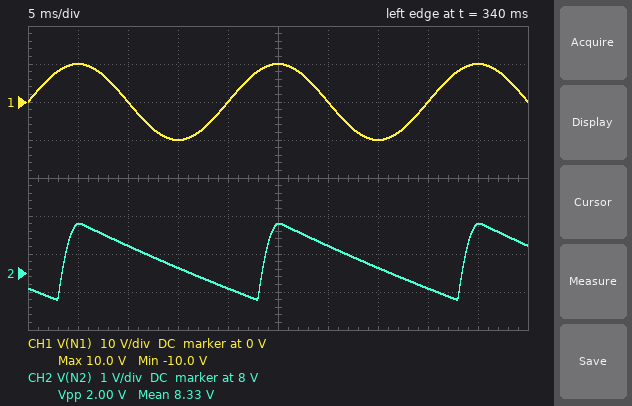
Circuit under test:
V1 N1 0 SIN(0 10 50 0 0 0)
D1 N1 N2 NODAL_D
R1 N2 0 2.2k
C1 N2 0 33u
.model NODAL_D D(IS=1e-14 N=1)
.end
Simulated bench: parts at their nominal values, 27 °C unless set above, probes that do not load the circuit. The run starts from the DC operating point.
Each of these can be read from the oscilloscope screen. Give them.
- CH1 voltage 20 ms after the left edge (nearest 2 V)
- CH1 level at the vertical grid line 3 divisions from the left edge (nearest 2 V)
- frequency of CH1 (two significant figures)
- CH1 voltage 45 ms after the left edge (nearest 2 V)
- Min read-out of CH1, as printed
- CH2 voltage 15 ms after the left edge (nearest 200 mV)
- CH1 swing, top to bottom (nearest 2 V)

0 V
-10 V
50 Hz
10 V
-10.0 V
8.2 V
20 V
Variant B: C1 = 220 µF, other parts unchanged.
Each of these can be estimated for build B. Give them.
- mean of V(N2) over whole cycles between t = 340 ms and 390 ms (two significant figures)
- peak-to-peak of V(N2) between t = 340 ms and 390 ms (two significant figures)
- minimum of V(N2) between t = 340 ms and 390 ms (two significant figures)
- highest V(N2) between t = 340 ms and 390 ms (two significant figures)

9.1 V
350 mV
8.9 V
9.3 V
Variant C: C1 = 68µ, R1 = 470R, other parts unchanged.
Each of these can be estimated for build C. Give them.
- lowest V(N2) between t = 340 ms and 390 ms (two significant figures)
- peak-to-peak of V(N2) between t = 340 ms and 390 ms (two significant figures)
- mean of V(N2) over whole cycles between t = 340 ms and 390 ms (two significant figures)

5.5 V
3.8 V
7.3 V
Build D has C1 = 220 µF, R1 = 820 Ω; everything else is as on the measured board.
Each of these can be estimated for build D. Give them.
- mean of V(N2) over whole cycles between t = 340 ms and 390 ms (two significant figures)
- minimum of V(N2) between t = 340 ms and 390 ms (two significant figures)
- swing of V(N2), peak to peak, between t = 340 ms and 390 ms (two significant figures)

8.8 V
8.4 V
890 mV
